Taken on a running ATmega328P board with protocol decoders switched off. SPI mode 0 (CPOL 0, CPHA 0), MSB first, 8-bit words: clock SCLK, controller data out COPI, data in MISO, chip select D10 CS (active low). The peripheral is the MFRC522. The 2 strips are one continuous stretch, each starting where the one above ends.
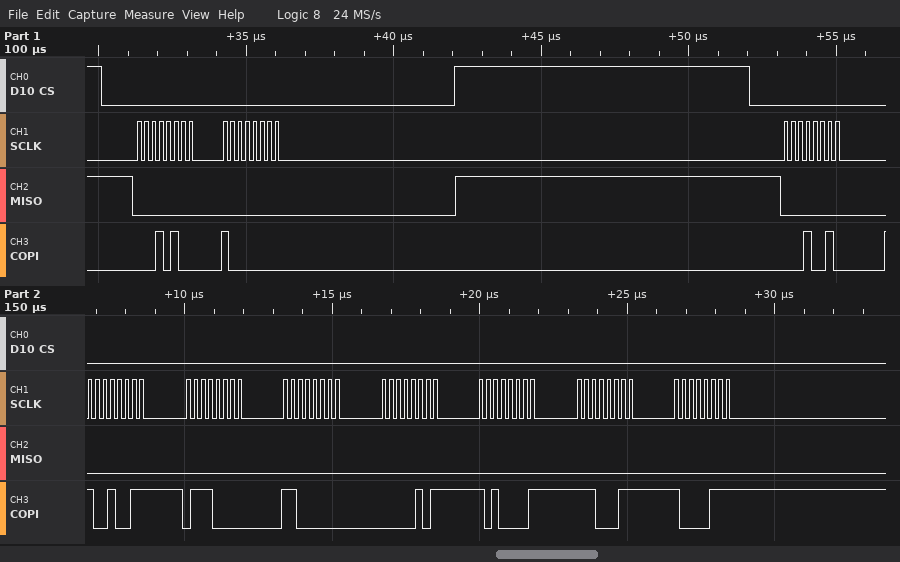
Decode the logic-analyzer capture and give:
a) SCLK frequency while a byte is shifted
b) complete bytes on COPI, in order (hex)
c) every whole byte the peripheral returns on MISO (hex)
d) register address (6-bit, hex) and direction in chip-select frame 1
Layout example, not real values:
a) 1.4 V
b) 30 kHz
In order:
a) 4 MHz
b) 14 80 12 93 70 C0 05 A1 E3 87
c) 00 00 00 00 00 00 00 00 00 00
d) 0x0A write
